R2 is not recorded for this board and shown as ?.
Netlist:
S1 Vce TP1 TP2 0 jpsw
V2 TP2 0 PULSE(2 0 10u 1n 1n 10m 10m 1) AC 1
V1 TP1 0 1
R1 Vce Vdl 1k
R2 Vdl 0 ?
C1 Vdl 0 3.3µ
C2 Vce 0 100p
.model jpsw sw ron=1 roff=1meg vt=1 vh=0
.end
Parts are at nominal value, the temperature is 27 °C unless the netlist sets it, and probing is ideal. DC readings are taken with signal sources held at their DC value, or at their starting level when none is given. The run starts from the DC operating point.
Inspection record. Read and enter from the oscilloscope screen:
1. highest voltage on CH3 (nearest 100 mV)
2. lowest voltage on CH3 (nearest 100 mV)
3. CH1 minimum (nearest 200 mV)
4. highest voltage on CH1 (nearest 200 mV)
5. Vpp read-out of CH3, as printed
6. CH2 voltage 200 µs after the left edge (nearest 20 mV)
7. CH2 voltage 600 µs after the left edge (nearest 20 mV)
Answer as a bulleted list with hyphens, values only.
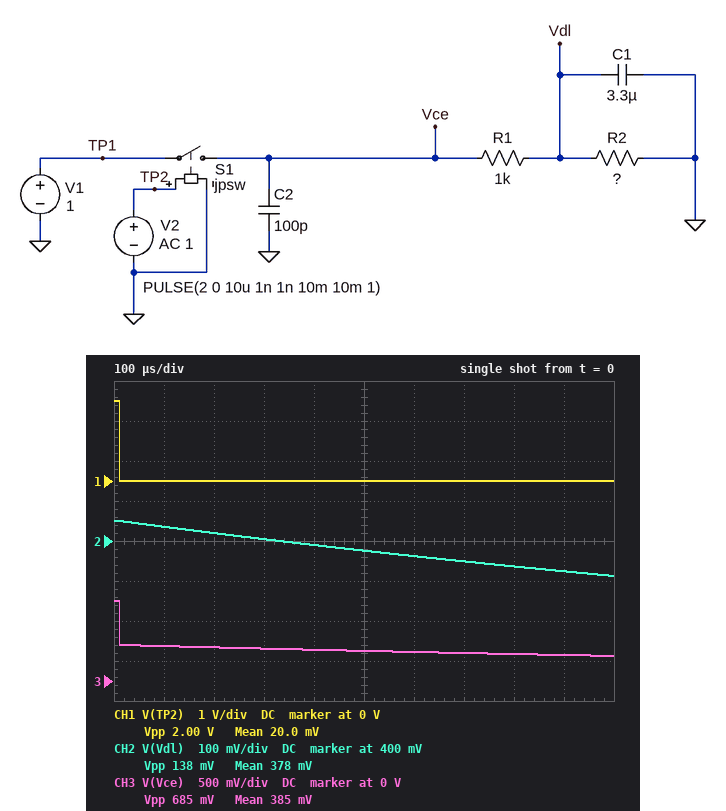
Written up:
- 1.0 V
- 300 mV
- 0 V
- 2.0 V
- 685 mV
- 420 mV
- 360 mV
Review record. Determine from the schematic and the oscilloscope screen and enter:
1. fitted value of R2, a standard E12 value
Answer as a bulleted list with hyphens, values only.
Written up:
- 820 Ω
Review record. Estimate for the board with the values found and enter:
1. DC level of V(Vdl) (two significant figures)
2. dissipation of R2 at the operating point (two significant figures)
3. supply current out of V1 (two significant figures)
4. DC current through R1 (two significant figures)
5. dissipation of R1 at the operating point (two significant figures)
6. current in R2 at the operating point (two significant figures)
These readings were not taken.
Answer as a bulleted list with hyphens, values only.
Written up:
- 450 mV
- 250 µW
- 550 µA
- 550 µA
- 300 µW
- 550 µA
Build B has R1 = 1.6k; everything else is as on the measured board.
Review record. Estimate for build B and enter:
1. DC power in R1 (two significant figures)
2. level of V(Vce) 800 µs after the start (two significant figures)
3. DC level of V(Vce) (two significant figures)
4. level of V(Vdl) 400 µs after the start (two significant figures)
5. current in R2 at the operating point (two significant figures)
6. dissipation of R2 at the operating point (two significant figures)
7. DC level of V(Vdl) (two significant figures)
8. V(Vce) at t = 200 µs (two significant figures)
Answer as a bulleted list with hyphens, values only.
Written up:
- 270 µW
- 250 mV
- 1.0 V
- 290 mV
- 410 µA
- 140 µW
- 340 mV
- 320 mV
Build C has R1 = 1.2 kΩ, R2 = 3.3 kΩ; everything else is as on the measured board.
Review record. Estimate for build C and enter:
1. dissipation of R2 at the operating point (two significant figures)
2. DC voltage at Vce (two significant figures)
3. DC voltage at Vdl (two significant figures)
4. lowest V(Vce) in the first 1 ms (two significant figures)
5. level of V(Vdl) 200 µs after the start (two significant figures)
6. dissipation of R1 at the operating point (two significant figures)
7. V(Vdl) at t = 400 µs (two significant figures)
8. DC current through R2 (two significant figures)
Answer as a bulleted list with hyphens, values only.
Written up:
- 160 µW
- 1.0 V
- 730 mV
- 670 mV
- 720 mV
- 59 µW
- 710 mV
- 220 µA
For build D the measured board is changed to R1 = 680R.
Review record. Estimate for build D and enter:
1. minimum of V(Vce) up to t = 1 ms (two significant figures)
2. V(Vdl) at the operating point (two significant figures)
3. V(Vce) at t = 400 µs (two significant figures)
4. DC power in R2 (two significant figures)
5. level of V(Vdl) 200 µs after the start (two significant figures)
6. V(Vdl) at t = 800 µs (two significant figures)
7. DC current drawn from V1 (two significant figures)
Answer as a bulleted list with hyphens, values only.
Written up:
- 380 mV
- 550 mV
- 470 mV
- 360 µW
- 510 mV
- 410 mV
- 670 µA
